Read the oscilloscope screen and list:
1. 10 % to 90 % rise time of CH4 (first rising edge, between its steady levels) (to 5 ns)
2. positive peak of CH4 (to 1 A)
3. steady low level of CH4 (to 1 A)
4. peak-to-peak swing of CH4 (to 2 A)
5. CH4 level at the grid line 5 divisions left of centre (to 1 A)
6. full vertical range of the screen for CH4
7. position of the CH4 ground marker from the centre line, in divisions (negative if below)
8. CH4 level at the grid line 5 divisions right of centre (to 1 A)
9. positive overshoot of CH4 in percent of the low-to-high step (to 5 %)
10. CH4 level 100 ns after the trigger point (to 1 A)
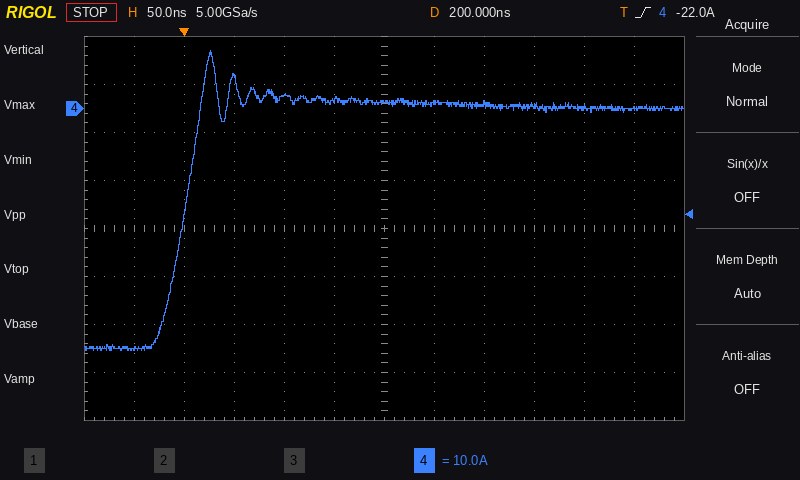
35 ns
12 A
-50 A
62 A
-50 A
80 A
+2.5 div
0 A
25 %
3 A
